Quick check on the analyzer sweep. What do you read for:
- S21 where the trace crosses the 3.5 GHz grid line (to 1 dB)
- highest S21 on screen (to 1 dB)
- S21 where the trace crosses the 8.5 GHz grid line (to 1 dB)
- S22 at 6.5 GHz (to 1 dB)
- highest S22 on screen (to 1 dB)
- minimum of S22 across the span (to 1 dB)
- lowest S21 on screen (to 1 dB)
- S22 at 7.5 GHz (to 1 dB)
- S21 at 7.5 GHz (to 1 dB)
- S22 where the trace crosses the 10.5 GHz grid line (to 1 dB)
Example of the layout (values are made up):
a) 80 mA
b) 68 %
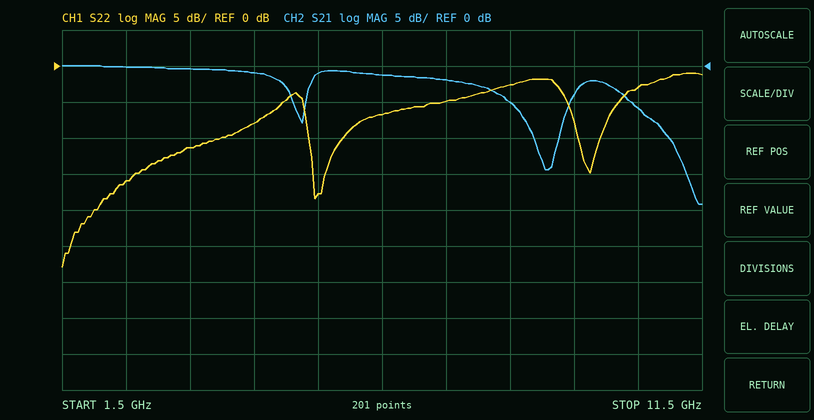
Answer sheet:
a) 0 dB
b) 0 dB
c) -5 dB
d) -7 dB
e) -1 dB
f) -28 dB
g) -19 dB
h) -5 dB
i) -2 dB
j) -3 dB
